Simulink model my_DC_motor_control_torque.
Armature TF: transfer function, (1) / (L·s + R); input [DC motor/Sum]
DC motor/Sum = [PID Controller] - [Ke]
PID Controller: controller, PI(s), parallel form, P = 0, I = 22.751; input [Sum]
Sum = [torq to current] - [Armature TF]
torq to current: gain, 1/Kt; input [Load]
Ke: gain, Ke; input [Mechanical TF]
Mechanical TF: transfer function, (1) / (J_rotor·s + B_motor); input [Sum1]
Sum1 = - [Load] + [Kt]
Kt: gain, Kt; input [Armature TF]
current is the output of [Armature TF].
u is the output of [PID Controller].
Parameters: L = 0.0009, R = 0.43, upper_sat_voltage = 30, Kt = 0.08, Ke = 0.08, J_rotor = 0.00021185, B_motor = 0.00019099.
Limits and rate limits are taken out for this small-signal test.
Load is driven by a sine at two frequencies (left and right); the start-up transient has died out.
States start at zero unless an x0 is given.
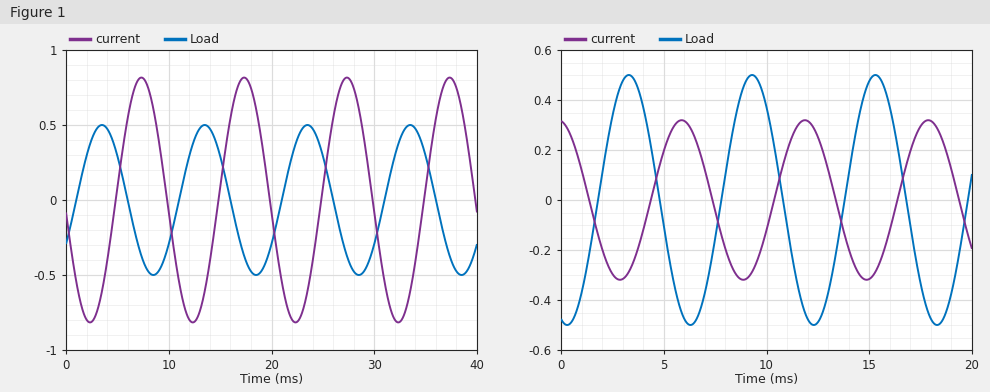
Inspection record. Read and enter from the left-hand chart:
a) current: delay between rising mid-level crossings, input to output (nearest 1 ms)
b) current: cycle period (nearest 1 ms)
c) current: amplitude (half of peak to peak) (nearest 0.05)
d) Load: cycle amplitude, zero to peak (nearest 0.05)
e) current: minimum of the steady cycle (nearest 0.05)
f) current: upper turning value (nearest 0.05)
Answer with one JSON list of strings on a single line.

["4 ms", "10 ms", "0.80", "0.50", "-0.80", "0.80"]
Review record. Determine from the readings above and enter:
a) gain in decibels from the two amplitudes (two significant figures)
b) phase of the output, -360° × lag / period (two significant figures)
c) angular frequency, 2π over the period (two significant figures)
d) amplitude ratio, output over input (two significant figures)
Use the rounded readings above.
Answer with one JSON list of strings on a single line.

["4.1 dB", "-140°", "0.63 rad/ms", "1.6"]
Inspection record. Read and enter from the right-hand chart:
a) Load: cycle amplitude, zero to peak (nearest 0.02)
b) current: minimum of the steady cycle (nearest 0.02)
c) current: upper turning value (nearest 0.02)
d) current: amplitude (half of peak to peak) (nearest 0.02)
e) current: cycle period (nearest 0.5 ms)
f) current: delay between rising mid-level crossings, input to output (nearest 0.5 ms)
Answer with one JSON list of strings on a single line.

["0.50", "-0.32", "0.32", "0.32", "6.0 ms", "2.5 ms"]
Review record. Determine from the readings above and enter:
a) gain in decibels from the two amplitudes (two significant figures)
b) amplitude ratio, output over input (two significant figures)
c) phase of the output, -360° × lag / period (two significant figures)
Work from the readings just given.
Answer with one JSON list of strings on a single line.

["-3.9 dB", "0.64", "-150°"]
